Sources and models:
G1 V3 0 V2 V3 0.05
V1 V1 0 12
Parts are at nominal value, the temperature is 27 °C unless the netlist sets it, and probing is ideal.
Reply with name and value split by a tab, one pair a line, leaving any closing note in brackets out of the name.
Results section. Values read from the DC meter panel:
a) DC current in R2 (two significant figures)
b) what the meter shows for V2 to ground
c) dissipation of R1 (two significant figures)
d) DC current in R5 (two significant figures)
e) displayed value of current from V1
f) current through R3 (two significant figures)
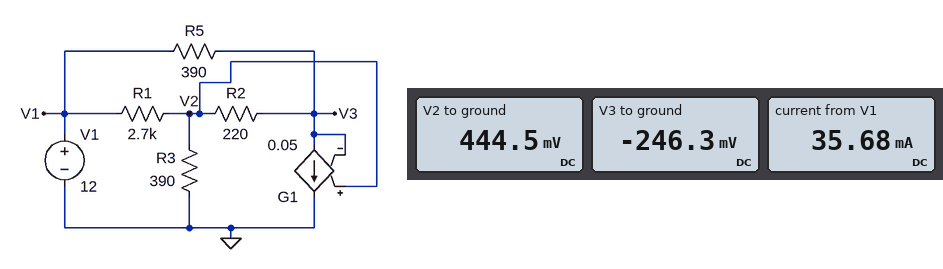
DC current in R2	3.1 mA
what the meter shows for V2 to ground	444.5 mV
dissipation of R1	49 mW
DC current in R5	31 mA
displayed value of current from V1	35.68 mA
current through R3	1.1 mA
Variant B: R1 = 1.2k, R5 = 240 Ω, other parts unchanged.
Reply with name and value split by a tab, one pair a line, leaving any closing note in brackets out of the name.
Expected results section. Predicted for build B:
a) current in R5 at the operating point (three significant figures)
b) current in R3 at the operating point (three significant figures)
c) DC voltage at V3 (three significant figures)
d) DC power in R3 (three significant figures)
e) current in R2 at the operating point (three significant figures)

current in R5 at the operating point	48.0 mA
current in R3 at the operating point	3.92 mA
DC voltage at V3	473 mV
DC power in R3	6.00 mW
current in R2 at the operating point	4.80 mA
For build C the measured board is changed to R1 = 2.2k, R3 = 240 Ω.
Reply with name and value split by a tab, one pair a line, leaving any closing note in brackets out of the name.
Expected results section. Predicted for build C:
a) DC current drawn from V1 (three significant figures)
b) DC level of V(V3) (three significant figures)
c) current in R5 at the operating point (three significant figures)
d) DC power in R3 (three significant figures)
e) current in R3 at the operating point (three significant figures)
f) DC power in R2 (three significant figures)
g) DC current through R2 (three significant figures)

DC current drawn from V1	36.5 mA
DC level of V(V3)	-183 mV
current in R5 at the operating point	31.2 mA
DC power in R3	1.06 mW
current in R3 at the operating point	2.10 mA
DC power in R2	2.15 mW
DC current through R2	3.12 mA
